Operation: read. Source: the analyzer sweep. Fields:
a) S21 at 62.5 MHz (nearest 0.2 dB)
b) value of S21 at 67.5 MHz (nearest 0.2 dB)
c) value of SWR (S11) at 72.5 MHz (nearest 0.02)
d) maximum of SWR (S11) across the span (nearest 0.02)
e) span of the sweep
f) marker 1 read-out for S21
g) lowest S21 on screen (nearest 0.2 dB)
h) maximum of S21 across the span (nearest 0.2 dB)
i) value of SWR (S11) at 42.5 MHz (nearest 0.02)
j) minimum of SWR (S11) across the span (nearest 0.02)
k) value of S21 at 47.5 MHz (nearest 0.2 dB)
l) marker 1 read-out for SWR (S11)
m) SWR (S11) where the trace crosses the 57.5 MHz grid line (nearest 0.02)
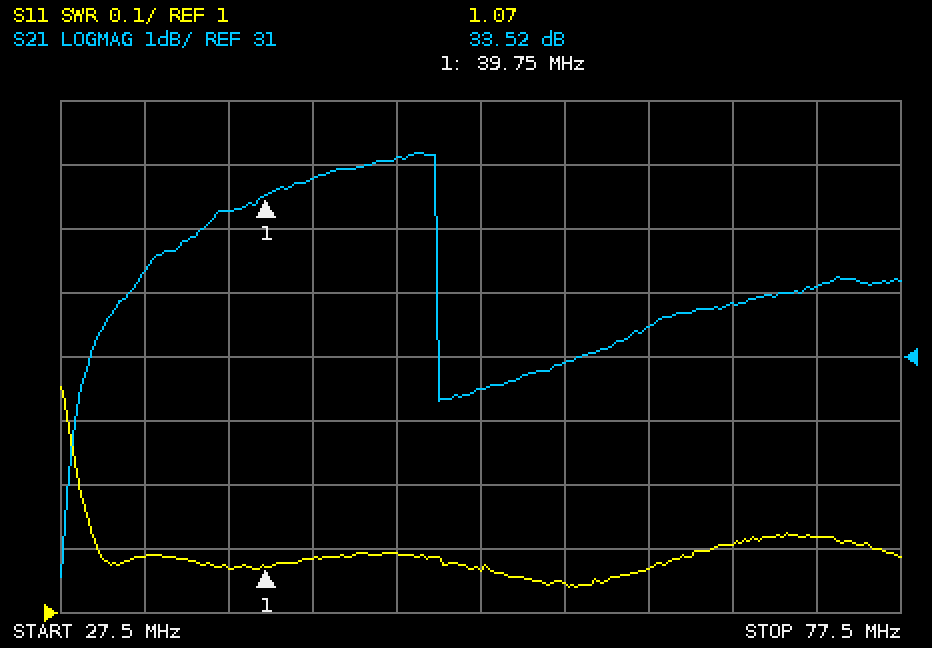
31.4 dB
31.8 dB
1.12
1.36
50 MHz
33.52 dB
27.6 dB
34.2 dB
1.08
1.04
34.2 dB
1.07
1.04
